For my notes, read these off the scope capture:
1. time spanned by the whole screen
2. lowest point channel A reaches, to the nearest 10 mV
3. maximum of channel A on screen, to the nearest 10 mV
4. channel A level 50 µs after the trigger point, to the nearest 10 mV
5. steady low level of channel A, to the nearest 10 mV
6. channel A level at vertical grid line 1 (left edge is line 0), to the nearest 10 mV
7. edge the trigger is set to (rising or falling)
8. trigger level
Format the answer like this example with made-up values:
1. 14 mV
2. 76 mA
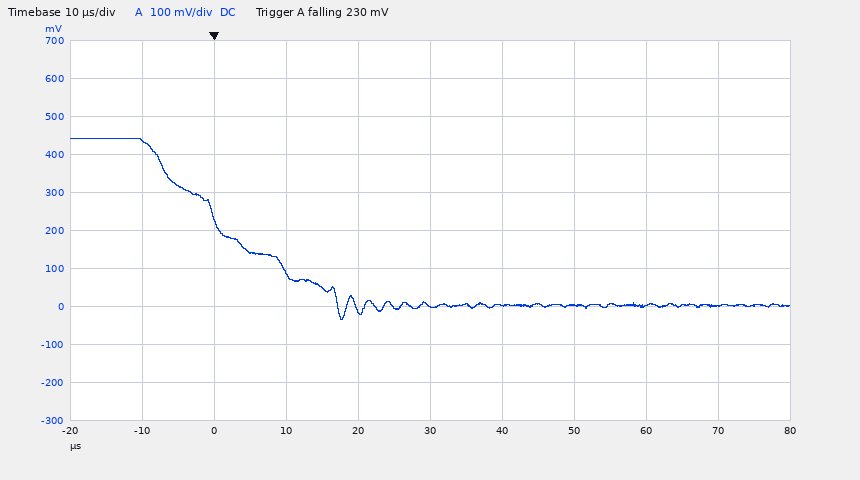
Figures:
1. 100 µs
2. -30 mV
3. 440 mV
4. 0 mV
5. 0 mV
6. 440 mV
7. falling
8. 230 mV
